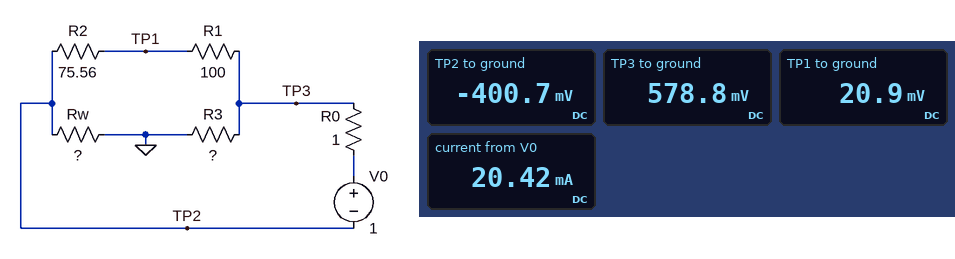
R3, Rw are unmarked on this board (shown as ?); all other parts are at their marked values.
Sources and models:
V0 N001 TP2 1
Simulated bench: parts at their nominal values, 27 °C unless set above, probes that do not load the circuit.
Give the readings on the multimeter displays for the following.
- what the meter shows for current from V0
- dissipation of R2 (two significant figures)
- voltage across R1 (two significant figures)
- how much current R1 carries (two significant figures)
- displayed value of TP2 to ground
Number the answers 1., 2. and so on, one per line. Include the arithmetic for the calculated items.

1. 20.42 mA
2. (20.9 mV - (-400.7 mV))^2 / 75.56 Ω = 2.4 mW
3. 578.8 mV - 20.9 mV = 560 mV
4. (578.8 mV - 20.9 mV) / 100 Ω = 5.6 mA
5. -400.7 mV
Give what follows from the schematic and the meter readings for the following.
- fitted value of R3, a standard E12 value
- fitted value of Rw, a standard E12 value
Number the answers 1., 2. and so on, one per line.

1. 39 Ω
2. 27 Ω
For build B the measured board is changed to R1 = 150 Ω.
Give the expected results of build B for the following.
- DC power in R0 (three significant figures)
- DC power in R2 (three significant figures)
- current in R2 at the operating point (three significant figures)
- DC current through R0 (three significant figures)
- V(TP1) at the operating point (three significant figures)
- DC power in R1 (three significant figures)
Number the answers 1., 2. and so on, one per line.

1. 369 µW
2. 1.43 mW
3. 4.35 mA
4. 19.2 mA
5. -72.7 mV
6. 2.84 mW
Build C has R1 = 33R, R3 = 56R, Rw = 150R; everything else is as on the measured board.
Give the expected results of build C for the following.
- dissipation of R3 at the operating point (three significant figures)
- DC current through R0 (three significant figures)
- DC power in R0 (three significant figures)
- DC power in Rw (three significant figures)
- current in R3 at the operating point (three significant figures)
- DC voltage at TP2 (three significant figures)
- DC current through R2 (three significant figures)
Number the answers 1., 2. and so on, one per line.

1. 1.28 mW
2. 13.9 mA
3. 192 µW
4. 3.44 mW
5. 4.79 mA
6. -718 mV
7. 9.08 mA
